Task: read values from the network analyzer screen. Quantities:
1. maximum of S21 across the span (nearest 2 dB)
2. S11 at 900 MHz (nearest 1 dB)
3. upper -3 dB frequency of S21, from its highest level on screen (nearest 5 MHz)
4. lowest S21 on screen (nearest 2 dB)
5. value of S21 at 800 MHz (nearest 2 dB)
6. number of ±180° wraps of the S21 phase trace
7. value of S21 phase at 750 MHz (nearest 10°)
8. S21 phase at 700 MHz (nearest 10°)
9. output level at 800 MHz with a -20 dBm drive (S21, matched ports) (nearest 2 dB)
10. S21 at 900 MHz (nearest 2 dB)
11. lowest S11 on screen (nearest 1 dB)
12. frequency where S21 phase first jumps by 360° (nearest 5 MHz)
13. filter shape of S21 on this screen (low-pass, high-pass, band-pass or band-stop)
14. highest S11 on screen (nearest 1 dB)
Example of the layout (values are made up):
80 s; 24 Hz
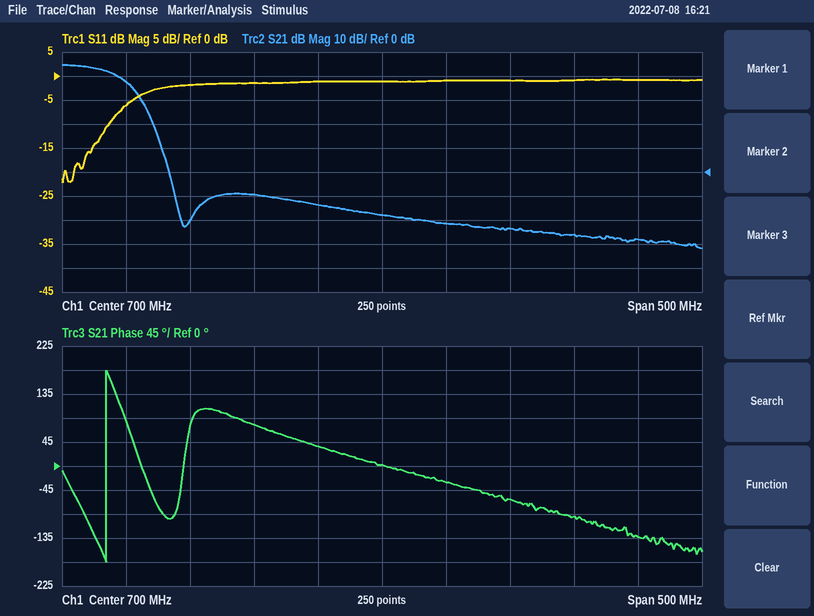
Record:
44 dB; -1 dB; 485 MHz; -32 dB; -24 dB; 1; -30°; 0°; -44 dBm; -28 dB; -22 dB; 485 MHz; low-pass; -1 dB
